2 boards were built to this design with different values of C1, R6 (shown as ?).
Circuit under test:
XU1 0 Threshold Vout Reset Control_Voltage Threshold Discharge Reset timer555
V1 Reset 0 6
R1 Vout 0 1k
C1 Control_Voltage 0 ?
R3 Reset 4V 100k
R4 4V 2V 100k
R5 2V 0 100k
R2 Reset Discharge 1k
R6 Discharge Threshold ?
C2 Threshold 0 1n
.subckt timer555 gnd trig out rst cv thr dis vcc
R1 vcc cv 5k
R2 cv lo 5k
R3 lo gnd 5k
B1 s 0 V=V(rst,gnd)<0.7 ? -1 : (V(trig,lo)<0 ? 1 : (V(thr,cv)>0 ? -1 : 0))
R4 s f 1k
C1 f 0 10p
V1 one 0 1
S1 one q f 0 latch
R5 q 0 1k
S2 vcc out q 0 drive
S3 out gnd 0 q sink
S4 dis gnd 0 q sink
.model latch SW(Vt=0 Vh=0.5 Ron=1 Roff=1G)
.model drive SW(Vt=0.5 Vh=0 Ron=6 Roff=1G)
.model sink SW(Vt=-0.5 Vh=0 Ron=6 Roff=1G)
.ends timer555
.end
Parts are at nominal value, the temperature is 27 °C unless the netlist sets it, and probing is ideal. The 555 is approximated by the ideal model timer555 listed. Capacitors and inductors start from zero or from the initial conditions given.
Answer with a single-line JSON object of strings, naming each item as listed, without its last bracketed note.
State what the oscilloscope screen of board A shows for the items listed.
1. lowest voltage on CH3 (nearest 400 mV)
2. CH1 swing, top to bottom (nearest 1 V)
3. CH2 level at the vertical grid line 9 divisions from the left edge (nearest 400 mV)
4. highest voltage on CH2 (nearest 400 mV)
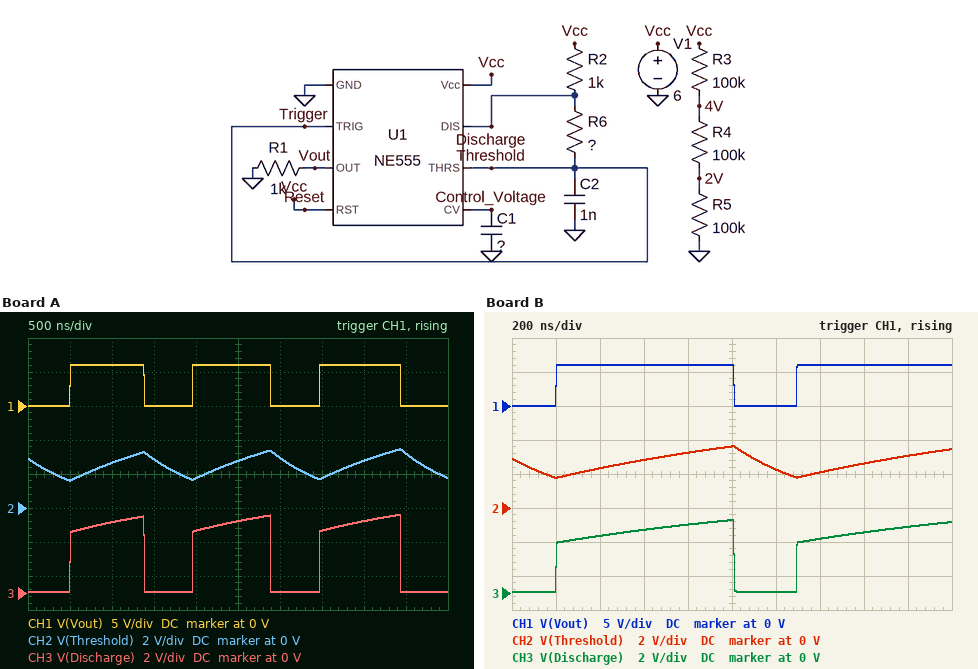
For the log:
{"lowest voltage on CH3": "0 V", "CH1 swing, top to bottom": "6 V", "CH2 level at the vertical grid line 9 divisions from the left edge": "3.2 V", "highest voltage on CH2": "3.6 V"}
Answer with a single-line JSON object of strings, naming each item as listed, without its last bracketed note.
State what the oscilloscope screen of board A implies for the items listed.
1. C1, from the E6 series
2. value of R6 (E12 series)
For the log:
{"C1, from the E6 series": "3.3 nF", "value of R6": "820 Ω"}
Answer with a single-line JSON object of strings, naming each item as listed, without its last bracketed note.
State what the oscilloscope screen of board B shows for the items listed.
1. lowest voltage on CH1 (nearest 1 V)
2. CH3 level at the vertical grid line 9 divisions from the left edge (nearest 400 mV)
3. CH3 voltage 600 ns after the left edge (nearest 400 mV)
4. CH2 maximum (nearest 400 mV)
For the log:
{"lowest voltage on CH1": "0 V", "CH3 level at the vertical grid line 9 divisions from the left edge": "4.0 V", "CH3 voltage 600 ns after the left edge": "3.6 V", "CH2 maximum": "3.6 V"}
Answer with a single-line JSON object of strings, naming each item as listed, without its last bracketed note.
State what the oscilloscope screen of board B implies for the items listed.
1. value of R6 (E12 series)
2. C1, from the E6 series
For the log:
{"value of R6": "390 Ω", "C1, from the E6 series": "3.3 nF"}
